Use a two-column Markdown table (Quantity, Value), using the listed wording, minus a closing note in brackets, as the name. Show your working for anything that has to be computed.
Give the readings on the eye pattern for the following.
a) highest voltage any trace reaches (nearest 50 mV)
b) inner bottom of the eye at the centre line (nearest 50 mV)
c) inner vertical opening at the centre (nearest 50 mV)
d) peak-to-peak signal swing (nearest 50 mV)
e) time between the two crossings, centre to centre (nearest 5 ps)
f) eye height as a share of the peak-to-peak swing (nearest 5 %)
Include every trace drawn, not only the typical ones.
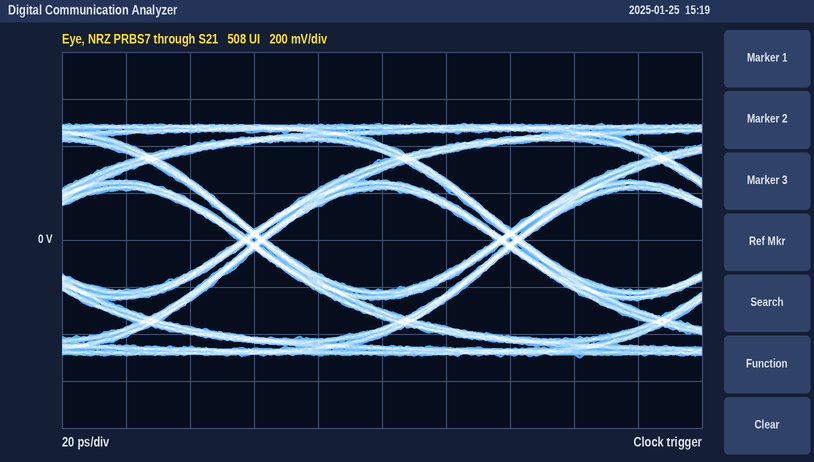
| Quantity | Value |
|---|---|
| highest voltage any trace reaches | 500 mV |
| inner bottom of the eye at the centre line | -200 mV |
| inner vertical opening at the centre | 450 mV |
| peak-to-peak signal swing | 1.00 V |
| time between the two crossings, centre to centre | 80 ps |
| eye height as a share of the peak-to-peak swing | 450 mV / 1.00 V ≈ 45 % |
